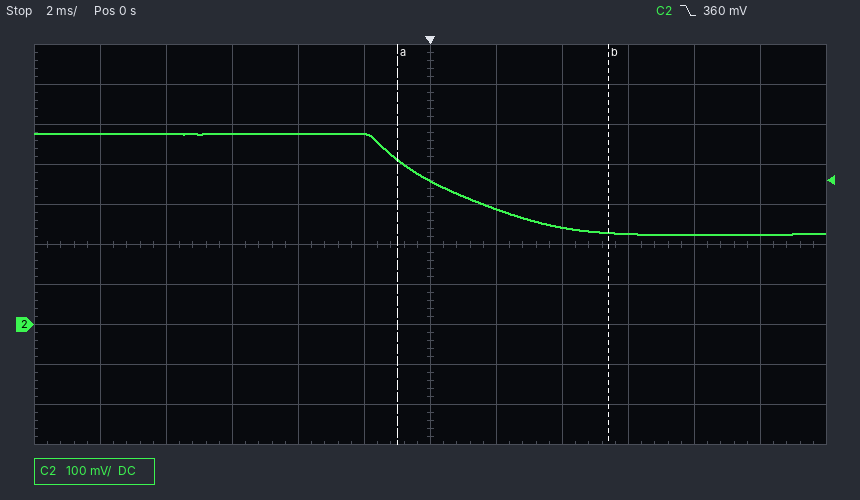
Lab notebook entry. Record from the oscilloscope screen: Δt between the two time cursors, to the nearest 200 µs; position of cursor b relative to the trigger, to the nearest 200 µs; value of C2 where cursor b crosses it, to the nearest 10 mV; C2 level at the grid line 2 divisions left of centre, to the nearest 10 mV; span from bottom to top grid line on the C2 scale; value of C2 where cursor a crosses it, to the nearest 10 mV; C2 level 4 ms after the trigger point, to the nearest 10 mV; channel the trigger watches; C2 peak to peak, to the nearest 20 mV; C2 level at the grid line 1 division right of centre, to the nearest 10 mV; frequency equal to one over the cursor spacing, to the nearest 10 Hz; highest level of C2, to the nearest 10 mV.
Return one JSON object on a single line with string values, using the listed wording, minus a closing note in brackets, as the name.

{"Δt between the two time cursors, to the nearest 200 µs": "6.4 ms", "position of cursor b relative to the trigger, to the nearest 200 µs": "+5.4 ms", "value of C2 where cursor b crosses it, to the nearest 10 mV": "230 mV", "C2 level at the grid line 2 divisions left of centre, to the nearest 10 mV": "480 mV", "span from bottom to top grid line on the C2 scale": "1 V", "value of C2 where cursor a crosses it, to the nearest 10 mV": "410 mV", "C2 level 4 ms after the trigger point, to the nearest 10 mV": "240 mV", "channel the trigger watches": "C2", "C2 peak to peak, to the nearest 20 mV": "260 mV", "C2 level at the grid line 1 division right of centre, to the nearest 10 mV": "290 mV", "frequency equal to one over the cursor spacing, to the nearest 10 Hz": "160 Hz", "highest level of C2, to the nearest 10 mV": "480 mV"}
